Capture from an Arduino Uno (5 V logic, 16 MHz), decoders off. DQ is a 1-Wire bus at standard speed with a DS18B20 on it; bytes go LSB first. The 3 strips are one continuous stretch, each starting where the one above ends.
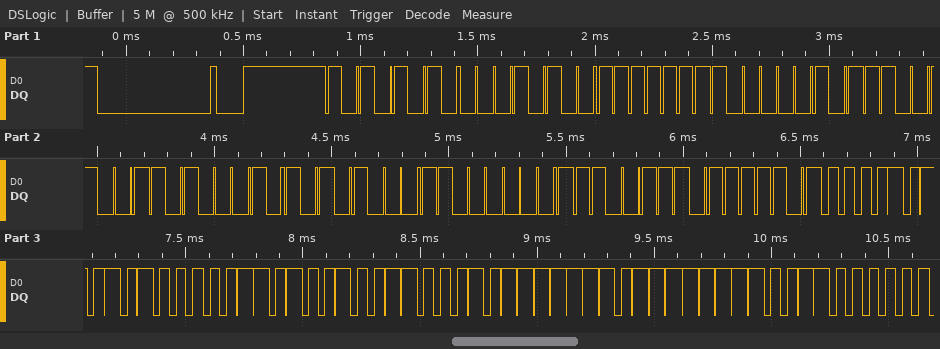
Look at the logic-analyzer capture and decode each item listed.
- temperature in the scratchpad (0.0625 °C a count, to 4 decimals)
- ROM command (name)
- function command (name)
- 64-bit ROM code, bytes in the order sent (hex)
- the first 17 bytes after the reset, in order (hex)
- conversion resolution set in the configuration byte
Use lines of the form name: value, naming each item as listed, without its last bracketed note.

temperature in the scratchpad: 85.0000 °C
ROM command: Match ROM
function command: Read Scratchpad
64-bit ROM code, bytes in the order sent: 28 FF A0 93 45 15 03 E7
the first 17 bytes after the reset, in order: 55 28 FF A0 93 45 15 03 E7 BE 50 05 4B 46 7F FF 0C
conversion resolution set in the configuration byte: 12 bits
